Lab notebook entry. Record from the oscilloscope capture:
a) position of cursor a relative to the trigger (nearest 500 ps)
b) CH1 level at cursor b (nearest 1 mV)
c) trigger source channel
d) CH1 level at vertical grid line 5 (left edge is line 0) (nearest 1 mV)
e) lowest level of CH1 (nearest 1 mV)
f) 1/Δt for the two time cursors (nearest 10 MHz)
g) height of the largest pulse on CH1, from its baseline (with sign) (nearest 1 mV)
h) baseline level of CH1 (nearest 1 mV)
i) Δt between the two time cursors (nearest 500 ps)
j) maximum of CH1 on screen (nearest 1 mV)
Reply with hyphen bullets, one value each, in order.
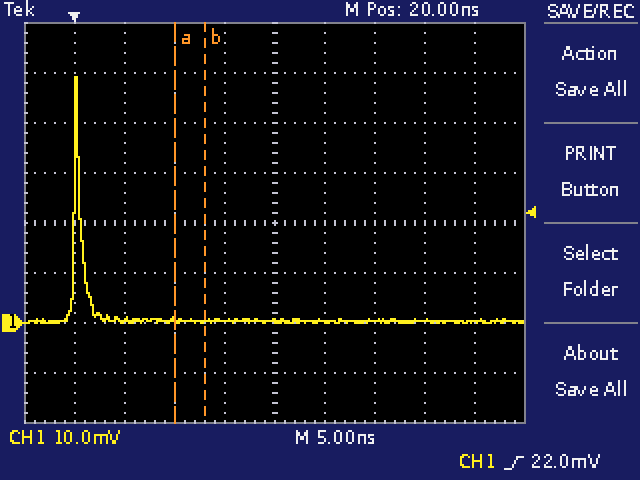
- +10.0 ns
- 0 mV
- CH1
- 0 mV
- 0 mV
- 330 MHz
- +49 mV
- 0 mV
- 3.0 ns
- 49 mV
